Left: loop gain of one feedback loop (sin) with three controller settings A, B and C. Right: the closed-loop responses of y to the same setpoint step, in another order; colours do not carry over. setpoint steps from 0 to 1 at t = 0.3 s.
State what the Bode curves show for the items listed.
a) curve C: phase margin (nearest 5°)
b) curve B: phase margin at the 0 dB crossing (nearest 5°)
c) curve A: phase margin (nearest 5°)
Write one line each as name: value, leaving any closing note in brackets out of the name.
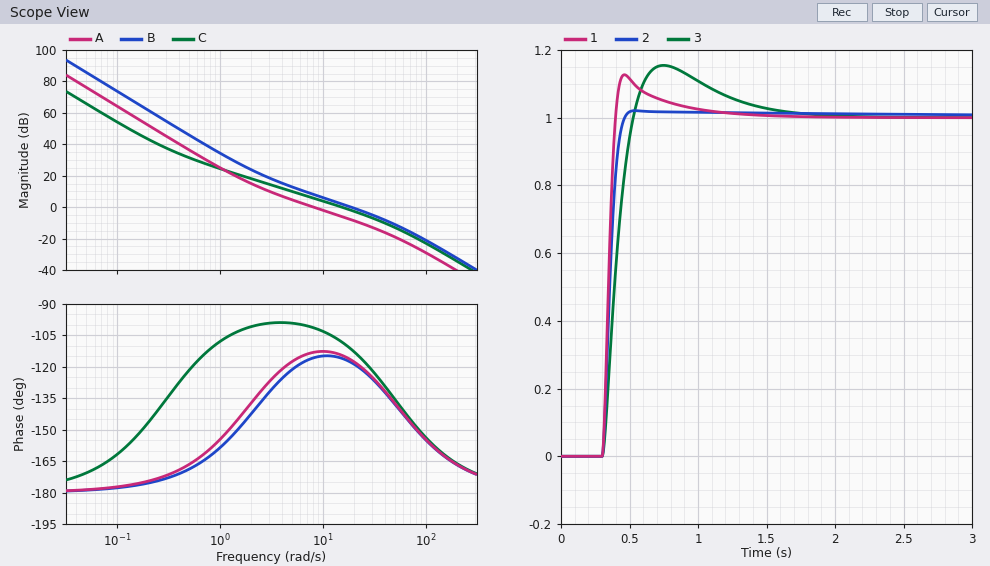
curve C: phase margin: 70°
curve B: phase margin at the 0 dB crossing: 60°
curve A: phase margin: 65°
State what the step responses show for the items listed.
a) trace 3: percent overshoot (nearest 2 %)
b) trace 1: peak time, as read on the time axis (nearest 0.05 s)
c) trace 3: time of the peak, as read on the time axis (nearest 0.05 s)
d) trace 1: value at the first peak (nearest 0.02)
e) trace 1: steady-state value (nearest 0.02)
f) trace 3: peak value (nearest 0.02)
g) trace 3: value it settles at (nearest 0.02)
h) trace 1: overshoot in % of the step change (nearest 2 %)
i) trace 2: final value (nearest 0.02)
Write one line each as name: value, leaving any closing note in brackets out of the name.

trace 3: percent overshoot: 16 %
trace 1: peak time, as read on the time axis: 0.45 s
trace 3: time of the peak, as read on the time axis: 0.75 s
trace 1: value at the first peak: 1.12
trace 1: steady-state value: 1.00
trace 3: peak value: 1.16
trace 3: value it settles at: 1.00
trace 1: overshoot in % of the step change: 12 %
trace 2: final value: 1.00
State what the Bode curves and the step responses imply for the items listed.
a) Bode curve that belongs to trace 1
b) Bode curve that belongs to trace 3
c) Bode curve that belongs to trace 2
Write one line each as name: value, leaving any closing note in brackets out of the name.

Bode curve that belongs to trace 1: B
Bode curve that belongs to trace 3: A
Bode curve that belongs to trace 2: C
